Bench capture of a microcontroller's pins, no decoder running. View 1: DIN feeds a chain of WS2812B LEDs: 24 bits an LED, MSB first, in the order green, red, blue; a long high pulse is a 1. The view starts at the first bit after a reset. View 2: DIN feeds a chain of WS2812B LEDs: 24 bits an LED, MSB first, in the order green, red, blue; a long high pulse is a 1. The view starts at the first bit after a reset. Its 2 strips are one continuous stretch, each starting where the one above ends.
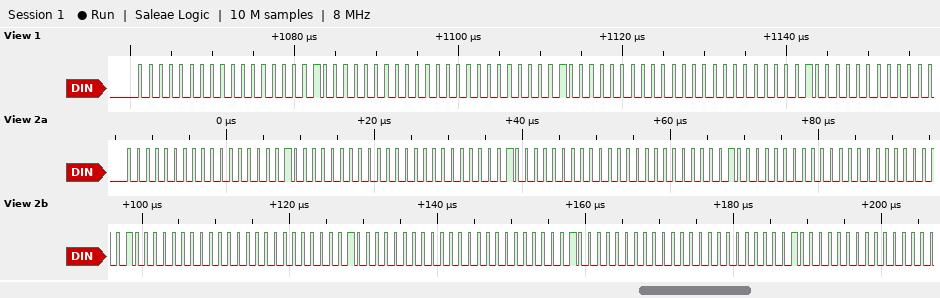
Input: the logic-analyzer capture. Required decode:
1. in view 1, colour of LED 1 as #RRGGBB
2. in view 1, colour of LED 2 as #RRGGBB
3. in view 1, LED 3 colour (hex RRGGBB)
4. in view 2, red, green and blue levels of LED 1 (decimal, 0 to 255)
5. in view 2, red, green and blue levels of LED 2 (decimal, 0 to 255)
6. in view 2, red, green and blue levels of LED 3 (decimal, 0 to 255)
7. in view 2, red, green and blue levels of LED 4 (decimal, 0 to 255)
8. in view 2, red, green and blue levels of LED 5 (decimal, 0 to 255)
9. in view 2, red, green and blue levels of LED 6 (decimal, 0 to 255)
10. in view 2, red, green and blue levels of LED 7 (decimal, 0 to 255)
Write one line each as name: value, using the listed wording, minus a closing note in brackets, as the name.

in view 1, colour of LED 1 as #RRGGBB: #000040
in view 1, colour of LED 2 as #RRGGBB: #000040
in view 1, LED 3 colour: #000040
in view 2, red, green and blue levels of LED 1: 0, 0, 64
in view 2, red, green and blue levels of LED 2: 0, 0, 64
in view 2, red, green and blue levels of LED 3: 0, 0, 64
in view 2, red, green and blue levels of LED 4: 0, 0, 64
in view 2, red, green and blue levels of LED 5: 0, 0, 64
in view 2, red, green and blue levels of LED 6: 0, 0, 64
in view 2, red, green and blue levels of LED 7: 0, 0, 64
